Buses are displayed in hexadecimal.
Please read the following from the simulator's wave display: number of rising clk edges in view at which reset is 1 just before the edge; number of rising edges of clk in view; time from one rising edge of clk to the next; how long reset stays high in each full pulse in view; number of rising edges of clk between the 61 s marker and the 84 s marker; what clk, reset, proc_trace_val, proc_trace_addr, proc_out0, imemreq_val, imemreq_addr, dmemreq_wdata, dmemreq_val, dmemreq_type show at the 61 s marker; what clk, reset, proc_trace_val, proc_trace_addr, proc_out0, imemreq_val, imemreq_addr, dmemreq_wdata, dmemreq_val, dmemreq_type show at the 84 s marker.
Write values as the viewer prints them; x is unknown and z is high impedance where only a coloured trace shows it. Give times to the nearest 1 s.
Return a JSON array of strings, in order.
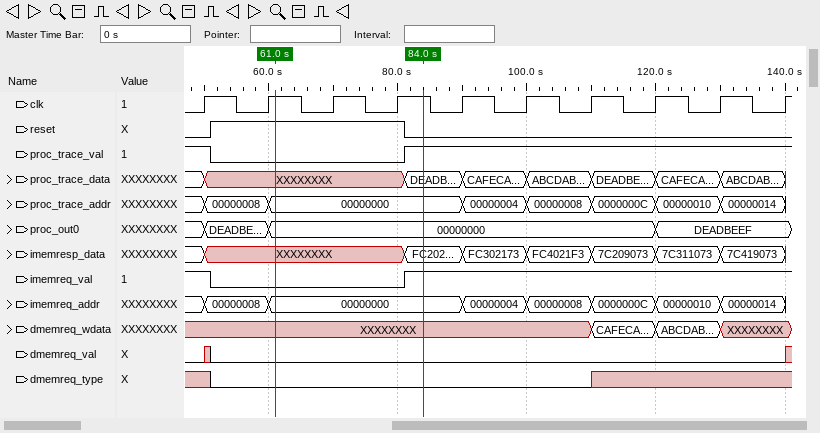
["3", "10", "10 s", "30 s", "2", "clk=1, reset=1, proc_trace_val=0, proc_trace_addr=00000000, proc_out0=00000000, imemreq_val=0, imemreq_addr=00000000, dmemreq_wdata=XXXXXXXX, dmemreq_val=0, dmemreq_type=0", "clk=1, reset=0, proc_trace_val=1, proc_trace_addr=00000000, proc_out0=00000000, imemreq_val=1, imemreq_addr=00000000, dmemreq_wdata=XXXXXXXX, dmemreq_val=0, dmemreq_type=0"]
